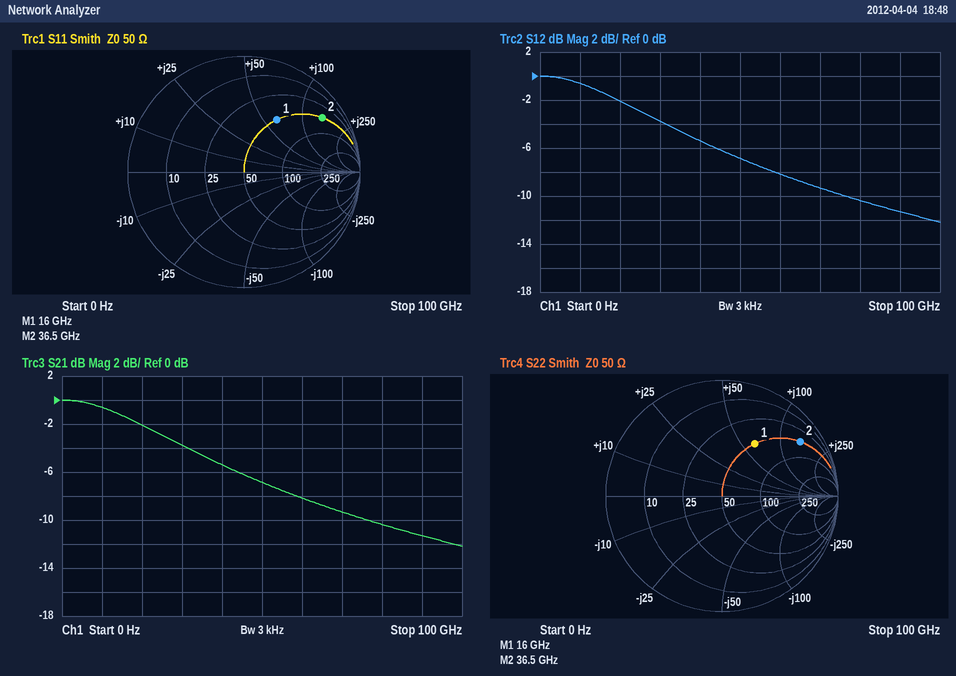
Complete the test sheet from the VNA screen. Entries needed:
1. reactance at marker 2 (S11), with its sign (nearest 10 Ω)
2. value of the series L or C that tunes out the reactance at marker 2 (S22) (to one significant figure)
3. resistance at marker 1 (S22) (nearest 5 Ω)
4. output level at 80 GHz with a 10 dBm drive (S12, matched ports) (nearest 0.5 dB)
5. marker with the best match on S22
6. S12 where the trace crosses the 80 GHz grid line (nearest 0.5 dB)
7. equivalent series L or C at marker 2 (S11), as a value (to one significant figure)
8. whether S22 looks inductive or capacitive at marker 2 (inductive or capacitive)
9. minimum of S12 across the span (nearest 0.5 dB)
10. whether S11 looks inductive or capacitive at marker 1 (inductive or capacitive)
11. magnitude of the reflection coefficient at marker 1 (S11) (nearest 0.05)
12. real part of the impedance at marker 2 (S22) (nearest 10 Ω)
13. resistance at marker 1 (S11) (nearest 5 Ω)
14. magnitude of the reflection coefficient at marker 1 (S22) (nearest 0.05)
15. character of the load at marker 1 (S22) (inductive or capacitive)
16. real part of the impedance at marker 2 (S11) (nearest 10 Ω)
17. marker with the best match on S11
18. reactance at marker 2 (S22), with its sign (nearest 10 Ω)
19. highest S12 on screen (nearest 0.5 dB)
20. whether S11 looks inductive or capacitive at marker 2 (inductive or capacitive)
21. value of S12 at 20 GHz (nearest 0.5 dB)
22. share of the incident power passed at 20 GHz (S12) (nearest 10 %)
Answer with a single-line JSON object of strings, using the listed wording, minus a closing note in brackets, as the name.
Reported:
{"reactance at marker 2 (S11), with its sign": "+140 Ω", "value of the series L or C that tunes out the reactance at marker 2 (S22)": "30 fF", "resistance at marker 1 (S22)": "50 Ω", "output level at 80 GHz with a 10 dBm drive (S12, matched ports)": "-0.5 dBm", "marker with the best match on S22": "marker 1", "S12 where the trace crosses the 80 GHz grid line": "-10.5 dB", "equivalent series L or C at marker 2 (S11), as a value": "600 pH", "whether S22 looks inductive or capacitive at marker 2": "inductive", "minimum of S12 across the span": "-12.0 dB", "whether S11 looks inductive or capacitive at marker 1": "inductive", "magnitude of the reflection coefficient at marker 1 (S11)": "0.55", "real part of the impedance at marker 2 (S22)": "50 Ω", "resistance at marker 1 (S11)": "50 Ω", "magnitude of the reflection coefficient at marker 1 (S22)": "0.55", "character of the load at marker 1 (S22)": "inductive", "real part of the impedance at marker 2 (S11)": "50 Ω", "marker with the best match on S11": "marker 1", "reactance at marker 2 (S22), with its sign": "+140 Ω", "highest S12 on screen": "0.0 dB", "whether S11 looks inductive or capacitive at marker 2": "inductive", "value of S12 at 20 GHz": "-2.0 dB", "share of the incident power passed at 20 GHz (S12)": "60 %"}
